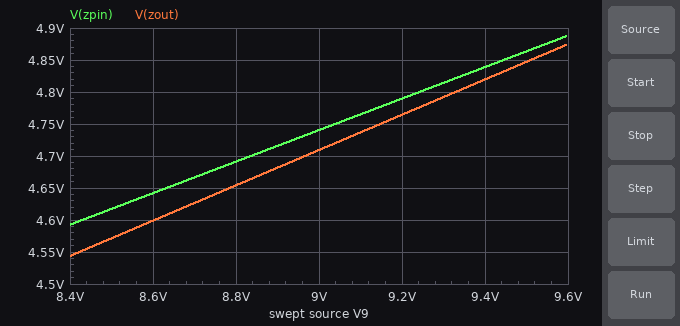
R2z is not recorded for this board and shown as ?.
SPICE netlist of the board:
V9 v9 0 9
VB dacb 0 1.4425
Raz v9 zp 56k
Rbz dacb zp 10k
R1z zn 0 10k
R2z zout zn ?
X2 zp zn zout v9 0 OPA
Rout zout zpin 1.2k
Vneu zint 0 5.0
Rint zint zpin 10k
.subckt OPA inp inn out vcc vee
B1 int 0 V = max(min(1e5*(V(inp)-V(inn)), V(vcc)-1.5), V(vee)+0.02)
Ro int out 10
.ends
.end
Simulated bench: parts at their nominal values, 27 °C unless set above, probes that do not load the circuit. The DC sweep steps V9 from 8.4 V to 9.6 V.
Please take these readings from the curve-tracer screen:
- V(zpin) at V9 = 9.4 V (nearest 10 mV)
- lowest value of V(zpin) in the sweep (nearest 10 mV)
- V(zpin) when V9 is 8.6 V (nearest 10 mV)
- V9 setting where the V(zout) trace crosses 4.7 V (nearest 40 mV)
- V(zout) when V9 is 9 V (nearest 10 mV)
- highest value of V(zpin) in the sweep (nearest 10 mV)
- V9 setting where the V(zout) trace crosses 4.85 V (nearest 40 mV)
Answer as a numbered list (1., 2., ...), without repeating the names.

1. 4.84 V
2. 4.59 V
3. 4.64 V
4. 8.96 V
5. 4.71 V
6. 4.89 V
7. 9.52 V
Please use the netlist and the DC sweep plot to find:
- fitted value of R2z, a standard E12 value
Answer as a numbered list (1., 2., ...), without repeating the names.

1. 8.2 kΩ
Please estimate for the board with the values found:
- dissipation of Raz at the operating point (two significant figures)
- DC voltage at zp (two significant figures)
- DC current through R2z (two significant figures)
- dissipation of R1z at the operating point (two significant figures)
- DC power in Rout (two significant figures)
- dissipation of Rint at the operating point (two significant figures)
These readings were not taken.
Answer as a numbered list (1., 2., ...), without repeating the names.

1. 730 µW
2. 2.6 V
3. 260 µA
4. 670 µW
5. 810 nW
6. 6.7 µW
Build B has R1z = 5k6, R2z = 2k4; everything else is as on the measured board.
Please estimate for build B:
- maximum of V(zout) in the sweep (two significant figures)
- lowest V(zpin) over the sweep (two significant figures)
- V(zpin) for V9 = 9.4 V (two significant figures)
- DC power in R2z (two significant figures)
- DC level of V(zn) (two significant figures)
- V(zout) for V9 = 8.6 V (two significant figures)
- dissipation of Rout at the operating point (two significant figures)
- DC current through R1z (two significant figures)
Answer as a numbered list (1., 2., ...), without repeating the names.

1. 3.8 V
2. 3.7 V
3. 3.9 V
4. 510 µW
5. 2.6 V
6. 3.6 V
7. 16 µW
8. 460 µA
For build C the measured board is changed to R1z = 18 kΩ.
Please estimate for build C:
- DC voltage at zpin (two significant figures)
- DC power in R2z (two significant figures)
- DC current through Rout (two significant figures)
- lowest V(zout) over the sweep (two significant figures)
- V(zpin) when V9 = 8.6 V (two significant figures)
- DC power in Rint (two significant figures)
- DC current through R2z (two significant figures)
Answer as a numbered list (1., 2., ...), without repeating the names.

1. 3.9 V
2. 170 µW
3. 110 µA
4. 3.6 V
5. 3.8 V
6. 120 µW
7. 140 µA
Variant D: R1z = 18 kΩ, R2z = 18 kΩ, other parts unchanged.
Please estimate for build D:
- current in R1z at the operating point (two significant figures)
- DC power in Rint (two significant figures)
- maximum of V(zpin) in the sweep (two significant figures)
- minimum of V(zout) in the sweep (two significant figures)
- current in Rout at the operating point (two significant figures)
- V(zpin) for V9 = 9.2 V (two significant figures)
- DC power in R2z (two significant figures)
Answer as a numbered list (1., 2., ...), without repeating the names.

1. 140 µA
2. 2.4 µW
3. 5.3 V
4. 5.0 V
5. 16 µA
6. 5.2 V
7. 370 µW
